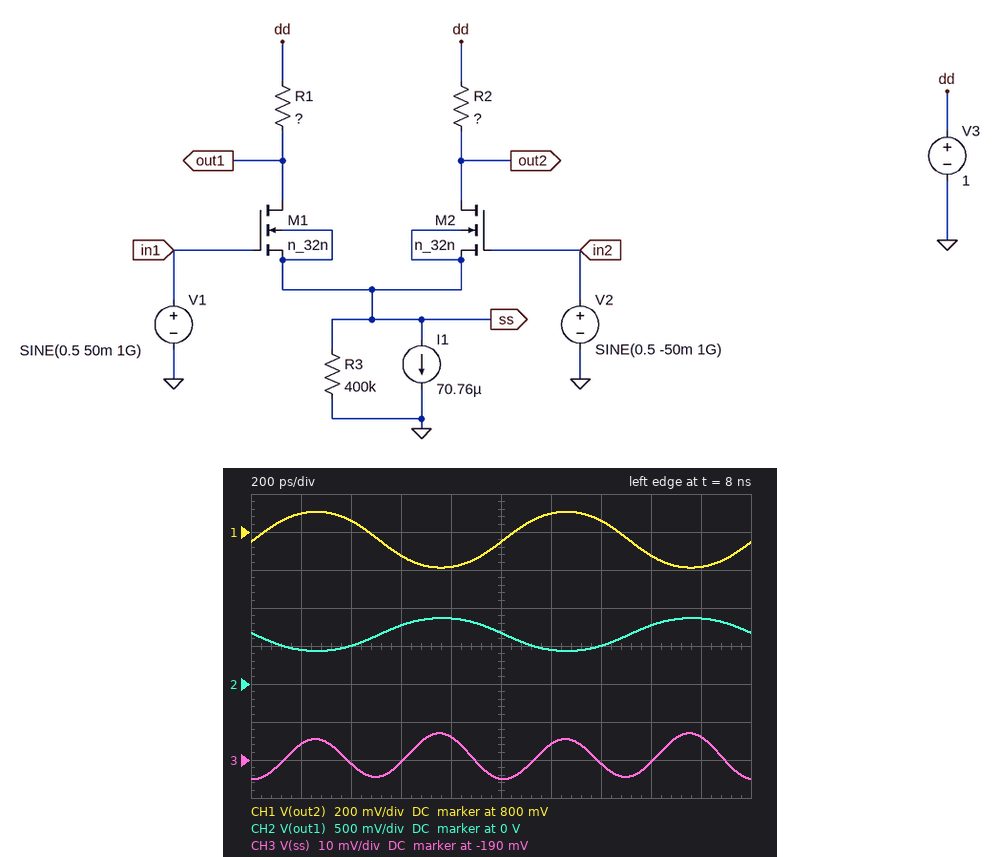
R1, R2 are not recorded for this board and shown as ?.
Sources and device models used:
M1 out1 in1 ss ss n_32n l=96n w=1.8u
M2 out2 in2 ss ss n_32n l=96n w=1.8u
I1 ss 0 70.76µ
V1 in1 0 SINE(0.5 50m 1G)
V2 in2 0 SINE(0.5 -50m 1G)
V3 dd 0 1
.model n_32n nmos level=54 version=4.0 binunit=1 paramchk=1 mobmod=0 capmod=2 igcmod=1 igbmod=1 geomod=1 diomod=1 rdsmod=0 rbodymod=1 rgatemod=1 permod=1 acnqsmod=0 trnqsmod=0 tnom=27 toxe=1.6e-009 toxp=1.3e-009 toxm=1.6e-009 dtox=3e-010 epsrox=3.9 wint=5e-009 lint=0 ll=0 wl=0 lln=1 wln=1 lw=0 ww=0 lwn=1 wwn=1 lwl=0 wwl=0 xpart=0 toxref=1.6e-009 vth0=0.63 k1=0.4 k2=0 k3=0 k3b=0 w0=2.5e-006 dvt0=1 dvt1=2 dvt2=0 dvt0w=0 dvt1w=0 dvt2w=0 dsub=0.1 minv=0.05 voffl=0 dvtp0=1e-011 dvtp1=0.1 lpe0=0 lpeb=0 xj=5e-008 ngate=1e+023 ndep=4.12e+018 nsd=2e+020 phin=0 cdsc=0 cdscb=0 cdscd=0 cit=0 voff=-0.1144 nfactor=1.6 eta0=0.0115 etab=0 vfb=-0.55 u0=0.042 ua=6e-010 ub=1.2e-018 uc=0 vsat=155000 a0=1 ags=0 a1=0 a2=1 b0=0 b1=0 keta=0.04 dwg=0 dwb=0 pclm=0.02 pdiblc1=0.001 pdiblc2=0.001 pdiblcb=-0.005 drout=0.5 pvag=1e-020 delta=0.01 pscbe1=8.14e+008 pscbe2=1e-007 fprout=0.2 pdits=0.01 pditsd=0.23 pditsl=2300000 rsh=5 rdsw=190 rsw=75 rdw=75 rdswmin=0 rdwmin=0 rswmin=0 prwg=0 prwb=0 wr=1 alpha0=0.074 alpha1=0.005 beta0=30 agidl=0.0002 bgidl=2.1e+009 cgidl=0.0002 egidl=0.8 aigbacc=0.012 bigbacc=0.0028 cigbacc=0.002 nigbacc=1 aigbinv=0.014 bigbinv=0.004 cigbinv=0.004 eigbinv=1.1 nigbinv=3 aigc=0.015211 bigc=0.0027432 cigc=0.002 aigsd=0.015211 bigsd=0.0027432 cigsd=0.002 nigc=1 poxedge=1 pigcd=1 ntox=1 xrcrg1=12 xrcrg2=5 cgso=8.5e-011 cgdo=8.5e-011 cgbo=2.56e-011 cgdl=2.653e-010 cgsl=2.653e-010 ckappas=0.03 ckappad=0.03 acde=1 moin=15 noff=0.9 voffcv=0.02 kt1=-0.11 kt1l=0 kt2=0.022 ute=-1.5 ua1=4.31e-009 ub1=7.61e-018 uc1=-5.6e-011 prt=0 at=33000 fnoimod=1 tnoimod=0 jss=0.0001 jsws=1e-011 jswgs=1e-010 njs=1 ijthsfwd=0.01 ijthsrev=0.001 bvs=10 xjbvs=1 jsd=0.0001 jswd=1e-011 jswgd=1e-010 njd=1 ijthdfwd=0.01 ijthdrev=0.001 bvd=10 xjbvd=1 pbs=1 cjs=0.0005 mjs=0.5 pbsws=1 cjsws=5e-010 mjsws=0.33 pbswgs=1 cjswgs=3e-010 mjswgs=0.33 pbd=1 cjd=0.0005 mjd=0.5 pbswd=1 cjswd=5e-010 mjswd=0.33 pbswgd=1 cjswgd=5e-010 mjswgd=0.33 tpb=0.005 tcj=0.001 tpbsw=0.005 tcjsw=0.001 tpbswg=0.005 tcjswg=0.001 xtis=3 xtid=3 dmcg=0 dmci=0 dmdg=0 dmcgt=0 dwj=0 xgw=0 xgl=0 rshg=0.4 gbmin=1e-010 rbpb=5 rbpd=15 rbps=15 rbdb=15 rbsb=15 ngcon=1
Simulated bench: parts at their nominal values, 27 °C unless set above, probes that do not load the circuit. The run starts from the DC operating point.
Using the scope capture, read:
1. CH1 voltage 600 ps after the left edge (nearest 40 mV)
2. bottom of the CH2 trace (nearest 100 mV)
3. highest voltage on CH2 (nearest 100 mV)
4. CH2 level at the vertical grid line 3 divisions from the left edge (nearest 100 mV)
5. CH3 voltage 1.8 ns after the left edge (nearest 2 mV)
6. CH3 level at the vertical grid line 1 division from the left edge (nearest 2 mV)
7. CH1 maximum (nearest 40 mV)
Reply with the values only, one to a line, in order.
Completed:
680 mV
400 mV
900 mV
800 mV
-184 mV
-186 mV
920 mV
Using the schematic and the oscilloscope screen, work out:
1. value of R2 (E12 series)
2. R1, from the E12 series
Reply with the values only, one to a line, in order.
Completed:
6.8 kΩ
10 kΩ
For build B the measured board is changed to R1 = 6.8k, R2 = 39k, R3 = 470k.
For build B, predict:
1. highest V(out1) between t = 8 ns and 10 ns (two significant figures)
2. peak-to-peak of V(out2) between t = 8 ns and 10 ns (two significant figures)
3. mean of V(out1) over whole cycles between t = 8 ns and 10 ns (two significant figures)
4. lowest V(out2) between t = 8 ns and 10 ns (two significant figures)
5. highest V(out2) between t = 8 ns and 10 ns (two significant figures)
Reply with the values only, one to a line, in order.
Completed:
750 mV
700 mV
690 mV
-220 mV
480 mV
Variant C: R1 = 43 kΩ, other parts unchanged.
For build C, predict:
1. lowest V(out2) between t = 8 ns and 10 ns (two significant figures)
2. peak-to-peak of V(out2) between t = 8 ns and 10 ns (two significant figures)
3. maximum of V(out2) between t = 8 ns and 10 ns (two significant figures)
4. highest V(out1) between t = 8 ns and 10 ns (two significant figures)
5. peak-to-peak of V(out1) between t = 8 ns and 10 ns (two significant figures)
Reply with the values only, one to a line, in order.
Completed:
610 mV
120 mV
730 mV
430 mV
660 mV
